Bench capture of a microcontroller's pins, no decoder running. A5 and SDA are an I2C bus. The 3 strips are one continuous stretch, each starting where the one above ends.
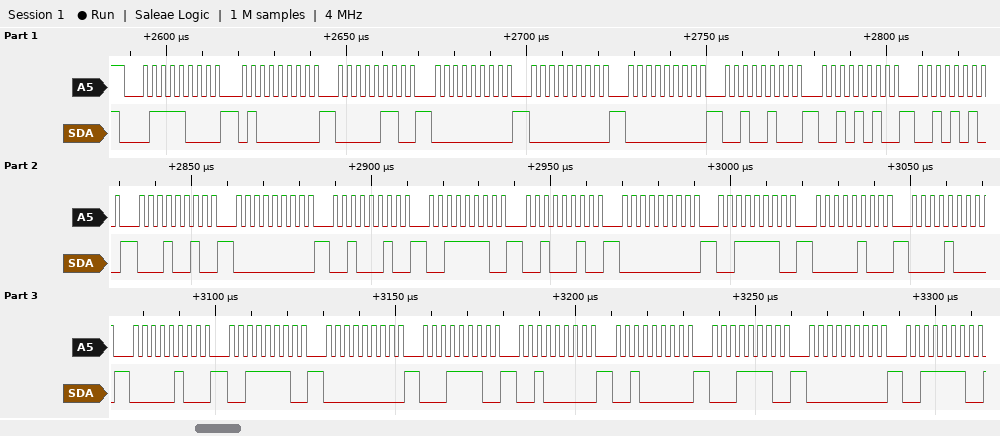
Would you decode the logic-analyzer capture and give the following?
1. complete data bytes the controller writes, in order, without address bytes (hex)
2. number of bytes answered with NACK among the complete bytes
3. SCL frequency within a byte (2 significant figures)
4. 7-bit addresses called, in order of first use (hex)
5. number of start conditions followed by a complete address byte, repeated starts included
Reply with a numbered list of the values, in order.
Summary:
1. 40 06 00 00 00 24 2A 2A 12 00 22 3E 22 00 3E 04 08 04 3E 00 1E 20 20 1E 00 3E
2. 0
3. 400 kHz
4. 0x3C
5. 1
